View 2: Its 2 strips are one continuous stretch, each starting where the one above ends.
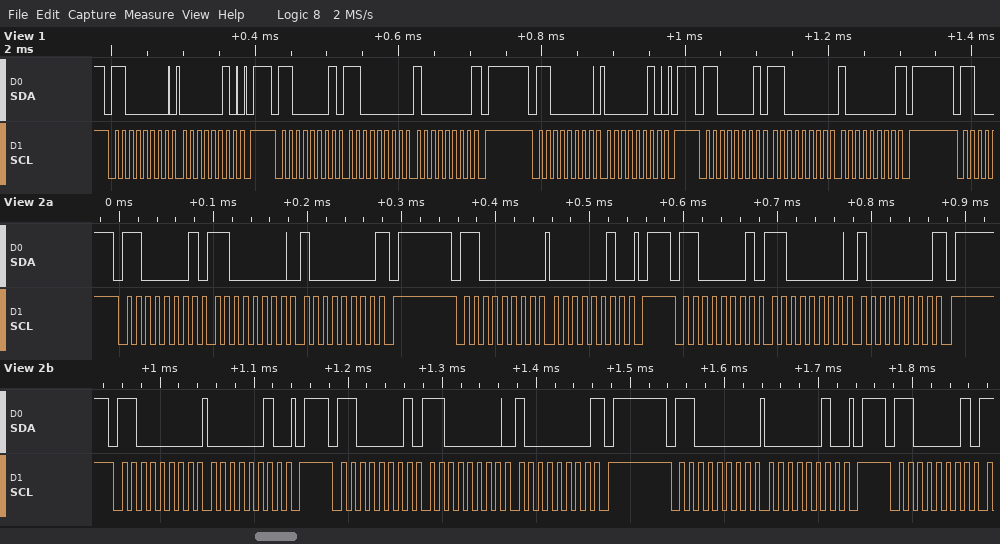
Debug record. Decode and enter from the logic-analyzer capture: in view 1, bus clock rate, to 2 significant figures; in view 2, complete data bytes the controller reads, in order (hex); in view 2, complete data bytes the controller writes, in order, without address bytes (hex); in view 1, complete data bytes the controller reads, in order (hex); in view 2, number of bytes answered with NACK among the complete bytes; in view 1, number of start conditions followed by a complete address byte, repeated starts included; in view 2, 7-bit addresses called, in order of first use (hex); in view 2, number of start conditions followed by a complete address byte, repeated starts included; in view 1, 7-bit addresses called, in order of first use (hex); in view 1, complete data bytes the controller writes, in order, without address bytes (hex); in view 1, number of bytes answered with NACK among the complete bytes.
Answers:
100 kHz
C0 80 C0 80 C0 80
02 02 02
C0 80 C0 80
3
4
0x60
7
0x60
02 02
2
